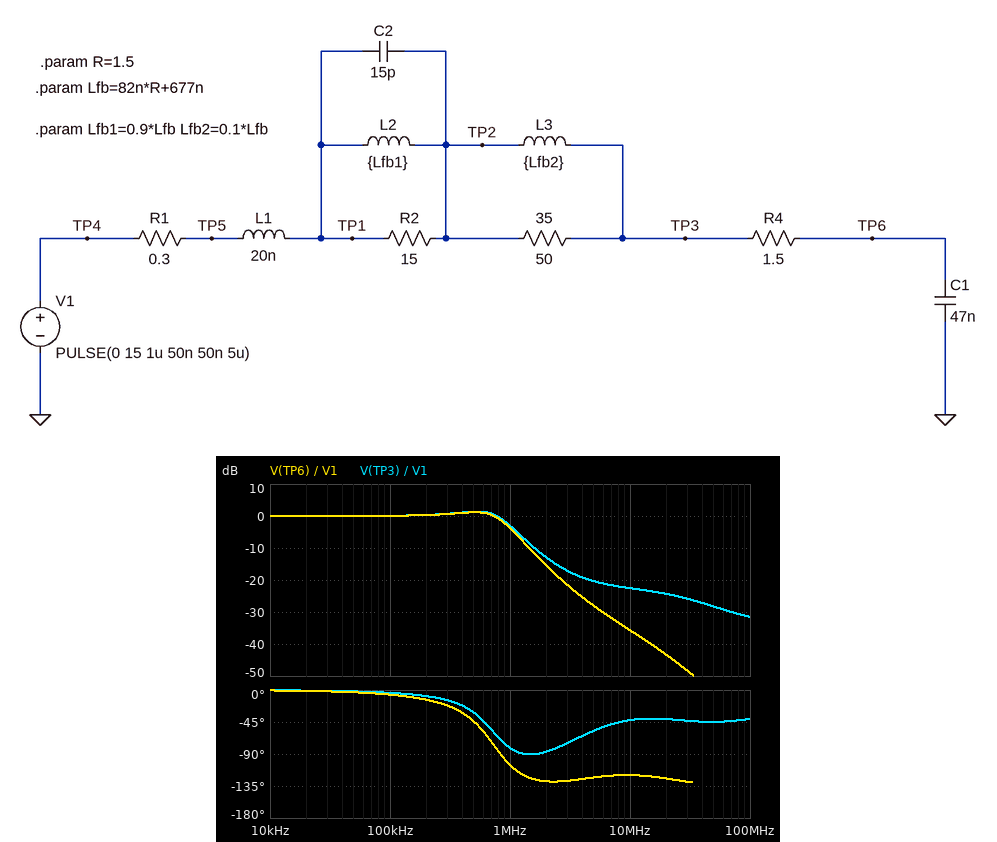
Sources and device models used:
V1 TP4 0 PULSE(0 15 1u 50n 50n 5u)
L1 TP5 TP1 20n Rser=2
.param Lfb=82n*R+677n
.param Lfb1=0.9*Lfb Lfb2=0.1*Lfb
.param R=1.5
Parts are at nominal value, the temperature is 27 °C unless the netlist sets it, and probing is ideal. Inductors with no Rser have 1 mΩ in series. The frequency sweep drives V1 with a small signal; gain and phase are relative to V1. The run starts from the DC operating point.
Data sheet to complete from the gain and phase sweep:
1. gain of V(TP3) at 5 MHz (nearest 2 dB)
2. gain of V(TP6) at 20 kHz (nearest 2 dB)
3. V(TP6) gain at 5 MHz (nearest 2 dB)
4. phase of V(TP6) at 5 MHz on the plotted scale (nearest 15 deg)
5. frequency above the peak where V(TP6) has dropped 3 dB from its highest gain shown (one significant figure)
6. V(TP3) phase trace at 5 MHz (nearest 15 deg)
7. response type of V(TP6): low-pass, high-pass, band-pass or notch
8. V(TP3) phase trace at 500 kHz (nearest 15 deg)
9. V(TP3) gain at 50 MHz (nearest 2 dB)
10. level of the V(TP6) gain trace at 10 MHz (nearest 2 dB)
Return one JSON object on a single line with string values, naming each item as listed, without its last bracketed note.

{"gain of V(TP3) at 5 MHz": "-20 dB", "gain of V(TP6) at 20 kHz": "0 dB", "V(TP6) gain at 5 MHz": "-28 dB", "phase of V(TP6) at 5 MHz on the plotted scale": "-120 deg", "frequency above the peak where V(TP6) has dropped 3 dB from its highest gain shown": "900 kHz", "V(TP3) phase trace at 5 MHz": "-60 deg", "response type of V(TP6): low-pass, high-pass, band-pass or notch": "low-pass", "V(TP3) phase trace at 500 kHz": "-30 deg", "V(TP3) gain at 50 MHz": "-28 dB", "level of the V(TP6) gain trace at 10 MHz": "-36 dB"}
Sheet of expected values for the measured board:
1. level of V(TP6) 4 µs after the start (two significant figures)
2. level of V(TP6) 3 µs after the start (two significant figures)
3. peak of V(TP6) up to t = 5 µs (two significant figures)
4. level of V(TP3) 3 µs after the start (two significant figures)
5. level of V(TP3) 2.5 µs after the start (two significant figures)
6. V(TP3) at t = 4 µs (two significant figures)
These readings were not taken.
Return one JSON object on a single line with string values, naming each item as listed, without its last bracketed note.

{"level of V(TP6) 4 µs after the start": "15 V", "level of V(TP6) 3 µs after the start": "15 V", "peak of V(TP6) up to t = 5 µs": "17 V", "level of V(TP3) 3 µs after the start": "15 V", "level of V(TP3) 2.5 µs after the start": "15 V", "V(TP3) at t = 4 µs": "15 V"}
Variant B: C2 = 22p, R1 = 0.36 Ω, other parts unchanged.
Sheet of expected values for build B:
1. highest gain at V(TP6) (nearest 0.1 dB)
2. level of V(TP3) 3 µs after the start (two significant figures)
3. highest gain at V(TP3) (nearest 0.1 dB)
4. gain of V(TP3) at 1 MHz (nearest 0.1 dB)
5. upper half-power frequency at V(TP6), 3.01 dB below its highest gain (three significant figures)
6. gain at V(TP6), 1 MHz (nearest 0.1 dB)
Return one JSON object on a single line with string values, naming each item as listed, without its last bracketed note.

{"highest gain at V(TP6)": "1.1 dB", "level of V(TP3) 3 µs after the start": "15 V", "highest gain at V(TP3)": "1.3 dB", "gain of V(TP3) at 1 MHz": "-3.1 dB", "upper half-power frequency at V(TP6), 3.01 dB below its highest gain": "871 kHz", "gain at V(TP6), 1 MHz": "-3.9 dB"}
